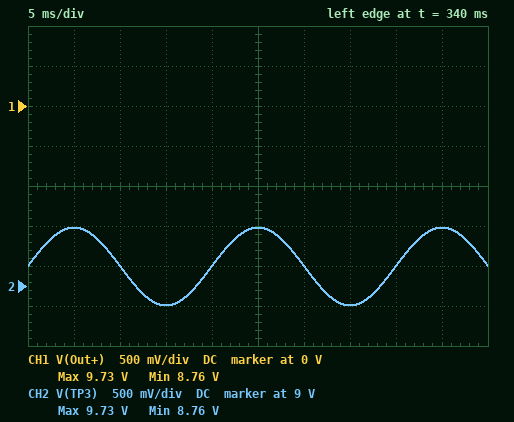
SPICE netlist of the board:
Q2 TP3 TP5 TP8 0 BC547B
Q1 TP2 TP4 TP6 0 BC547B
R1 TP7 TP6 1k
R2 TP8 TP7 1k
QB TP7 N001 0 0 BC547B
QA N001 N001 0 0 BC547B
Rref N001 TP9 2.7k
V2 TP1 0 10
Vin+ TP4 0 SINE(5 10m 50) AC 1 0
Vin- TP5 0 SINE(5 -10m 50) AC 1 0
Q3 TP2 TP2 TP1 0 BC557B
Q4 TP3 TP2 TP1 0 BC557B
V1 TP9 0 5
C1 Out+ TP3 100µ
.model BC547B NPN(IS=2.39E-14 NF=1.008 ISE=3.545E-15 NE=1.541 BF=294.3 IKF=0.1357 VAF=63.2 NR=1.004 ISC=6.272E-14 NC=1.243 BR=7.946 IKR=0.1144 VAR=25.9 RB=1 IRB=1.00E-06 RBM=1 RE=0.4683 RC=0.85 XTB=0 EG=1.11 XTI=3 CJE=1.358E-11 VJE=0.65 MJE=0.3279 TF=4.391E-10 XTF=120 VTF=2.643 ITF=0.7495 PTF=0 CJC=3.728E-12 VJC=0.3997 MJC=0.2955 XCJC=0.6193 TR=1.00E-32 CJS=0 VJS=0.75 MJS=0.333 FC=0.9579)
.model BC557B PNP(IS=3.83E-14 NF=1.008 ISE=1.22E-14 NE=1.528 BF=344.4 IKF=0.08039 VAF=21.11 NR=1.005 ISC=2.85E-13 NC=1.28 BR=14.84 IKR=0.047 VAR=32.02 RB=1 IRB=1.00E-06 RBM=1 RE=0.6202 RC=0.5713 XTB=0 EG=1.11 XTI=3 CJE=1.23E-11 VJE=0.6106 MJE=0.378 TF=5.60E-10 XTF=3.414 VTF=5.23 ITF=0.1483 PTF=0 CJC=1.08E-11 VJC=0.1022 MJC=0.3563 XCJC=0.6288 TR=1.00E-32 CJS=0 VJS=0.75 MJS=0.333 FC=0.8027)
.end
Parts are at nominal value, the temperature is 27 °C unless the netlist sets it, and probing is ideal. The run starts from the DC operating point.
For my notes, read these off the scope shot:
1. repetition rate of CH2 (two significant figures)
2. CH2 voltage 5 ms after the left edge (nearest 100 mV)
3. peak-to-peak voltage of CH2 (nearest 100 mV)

50 Hz
9.7 V
1.0 V
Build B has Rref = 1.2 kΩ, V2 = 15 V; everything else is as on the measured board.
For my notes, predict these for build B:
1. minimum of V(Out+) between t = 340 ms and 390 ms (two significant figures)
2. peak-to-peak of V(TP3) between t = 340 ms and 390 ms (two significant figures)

14 V
460 mV
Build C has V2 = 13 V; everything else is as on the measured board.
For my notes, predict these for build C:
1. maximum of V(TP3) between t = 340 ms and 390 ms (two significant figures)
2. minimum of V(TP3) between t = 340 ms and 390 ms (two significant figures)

13 V
12 V
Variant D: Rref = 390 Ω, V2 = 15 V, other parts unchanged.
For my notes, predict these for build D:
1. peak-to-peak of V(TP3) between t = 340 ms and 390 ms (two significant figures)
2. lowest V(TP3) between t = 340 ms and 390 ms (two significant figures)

210 mV
14 V
